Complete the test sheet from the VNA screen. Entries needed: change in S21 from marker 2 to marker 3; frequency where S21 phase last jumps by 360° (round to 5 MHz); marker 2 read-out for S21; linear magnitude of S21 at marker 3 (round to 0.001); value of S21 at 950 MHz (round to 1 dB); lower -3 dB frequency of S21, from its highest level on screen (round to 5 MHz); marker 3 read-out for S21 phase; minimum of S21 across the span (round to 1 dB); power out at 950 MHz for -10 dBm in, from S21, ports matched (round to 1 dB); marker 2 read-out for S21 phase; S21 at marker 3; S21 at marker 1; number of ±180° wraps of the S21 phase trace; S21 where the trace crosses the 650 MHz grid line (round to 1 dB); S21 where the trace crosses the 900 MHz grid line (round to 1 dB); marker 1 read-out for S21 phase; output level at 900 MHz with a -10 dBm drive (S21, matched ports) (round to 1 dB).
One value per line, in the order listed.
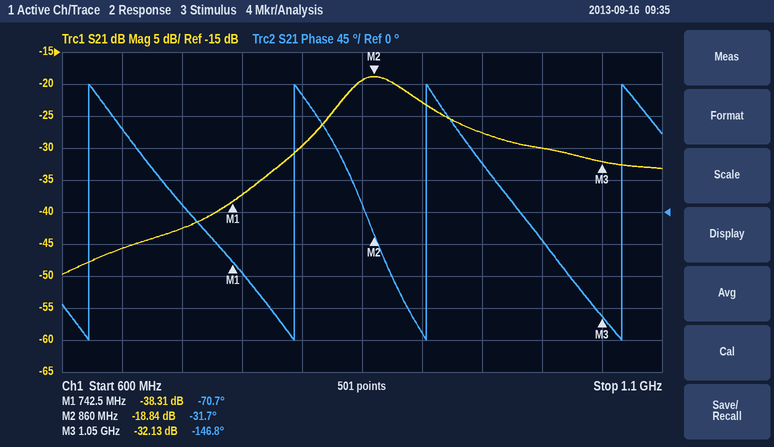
-13.29 dB
1.065 GHz
-18.84 dB
0.025
-28 dB
835 MHz
-146.8°
-50 dB
-38 dBm
-31.7°
-32.13 dB
-38.31 dB
4
-46 dB
-23 dB
-70.7°
-33 dBm
